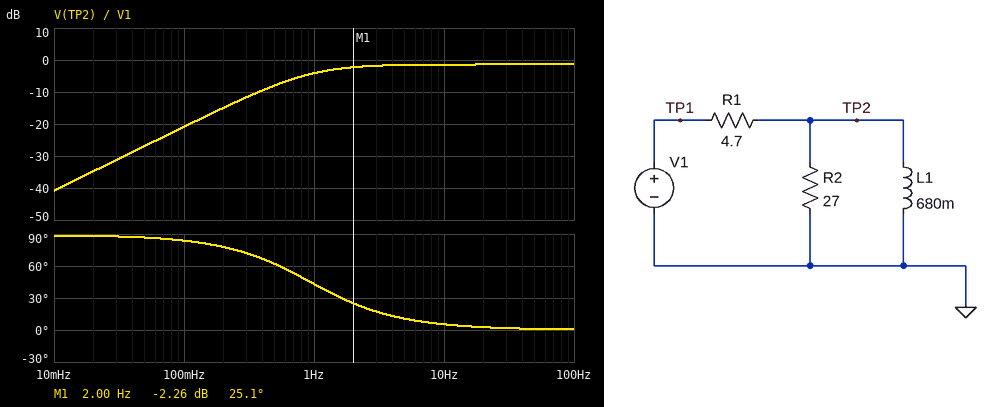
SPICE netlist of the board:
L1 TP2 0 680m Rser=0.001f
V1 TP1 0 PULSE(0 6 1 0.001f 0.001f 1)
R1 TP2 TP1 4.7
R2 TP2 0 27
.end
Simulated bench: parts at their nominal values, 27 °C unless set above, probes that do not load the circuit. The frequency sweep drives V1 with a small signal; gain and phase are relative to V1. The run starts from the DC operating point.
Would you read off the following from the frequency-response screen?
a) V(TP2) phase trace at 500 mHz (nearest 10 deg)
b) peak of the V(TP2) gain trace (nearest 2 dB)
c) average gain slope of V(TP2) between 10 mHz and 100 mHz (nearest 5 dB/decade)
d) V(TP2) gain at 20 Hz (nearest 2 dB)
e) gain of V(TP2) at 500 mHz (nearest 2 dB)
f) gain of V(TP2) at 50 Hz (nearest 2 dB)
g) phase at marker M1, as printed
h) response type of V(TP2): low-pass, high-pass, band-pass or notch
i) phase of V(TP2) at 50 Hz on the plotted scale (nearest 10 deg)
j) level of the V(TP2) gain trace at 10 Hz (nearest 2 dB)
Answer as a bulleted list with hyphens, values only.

- 60 deg
- -2 dB
- 20 dB/decade
- -2 dB
- -8 dB
- -2 dB
- 25.1 deg
- high-pass
- 0 deg
- -2 dB
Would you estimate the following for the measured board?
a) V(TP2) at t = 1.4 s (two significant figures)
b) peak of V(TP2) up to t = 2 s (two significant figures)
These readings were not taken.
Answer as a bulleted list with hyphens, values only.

- 490 mV
- 5.1 V
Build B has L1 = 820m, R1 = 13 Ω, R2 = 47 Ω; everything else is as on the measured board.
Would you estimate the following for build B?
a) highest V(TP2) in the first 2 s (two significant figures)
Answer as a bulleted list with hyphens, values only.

- 4.7 V
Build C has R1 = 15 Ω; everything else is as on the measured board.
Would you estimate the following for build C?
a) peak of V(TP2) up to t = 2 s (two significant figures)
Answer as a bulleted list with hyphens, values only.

- 3.9 V
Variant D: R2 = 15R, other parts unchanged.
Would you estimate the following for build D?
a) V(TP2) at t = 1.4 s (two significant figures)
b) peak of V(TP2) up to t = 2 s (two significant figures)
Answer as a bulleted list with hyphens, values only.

- 560 mV
- 4.6 V
